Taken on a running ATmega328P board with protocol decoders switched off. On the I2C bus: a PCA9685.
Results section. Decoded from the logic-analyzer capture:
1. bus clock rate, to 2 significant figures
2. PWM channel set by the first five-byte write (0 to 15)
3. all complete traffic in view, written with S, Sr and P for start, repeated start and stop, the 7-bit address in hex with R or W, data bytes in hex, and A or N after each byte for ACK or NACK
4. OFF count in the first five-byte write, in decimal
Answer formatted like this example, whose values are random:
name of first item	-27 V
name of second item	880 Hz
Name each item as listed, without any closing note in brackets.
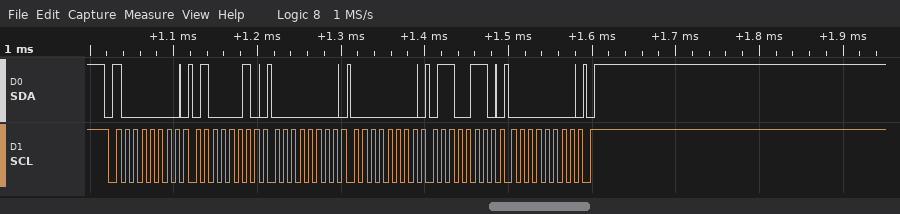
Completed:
bus clock rate, to 2 significant figures	100 kHz
PWM channel set by the first five-byte write	15
all complete traffic in view, written with S, Sr and P for start, repeated start and stop, the 7-bit address in hex with R or W, data bytes in hex, and A or N after each byte for ACK or NACK	S 40W A 42 A 00 A 00 A 66 A 00 A P
OFF count in the first five-byte write, in decimal	102
